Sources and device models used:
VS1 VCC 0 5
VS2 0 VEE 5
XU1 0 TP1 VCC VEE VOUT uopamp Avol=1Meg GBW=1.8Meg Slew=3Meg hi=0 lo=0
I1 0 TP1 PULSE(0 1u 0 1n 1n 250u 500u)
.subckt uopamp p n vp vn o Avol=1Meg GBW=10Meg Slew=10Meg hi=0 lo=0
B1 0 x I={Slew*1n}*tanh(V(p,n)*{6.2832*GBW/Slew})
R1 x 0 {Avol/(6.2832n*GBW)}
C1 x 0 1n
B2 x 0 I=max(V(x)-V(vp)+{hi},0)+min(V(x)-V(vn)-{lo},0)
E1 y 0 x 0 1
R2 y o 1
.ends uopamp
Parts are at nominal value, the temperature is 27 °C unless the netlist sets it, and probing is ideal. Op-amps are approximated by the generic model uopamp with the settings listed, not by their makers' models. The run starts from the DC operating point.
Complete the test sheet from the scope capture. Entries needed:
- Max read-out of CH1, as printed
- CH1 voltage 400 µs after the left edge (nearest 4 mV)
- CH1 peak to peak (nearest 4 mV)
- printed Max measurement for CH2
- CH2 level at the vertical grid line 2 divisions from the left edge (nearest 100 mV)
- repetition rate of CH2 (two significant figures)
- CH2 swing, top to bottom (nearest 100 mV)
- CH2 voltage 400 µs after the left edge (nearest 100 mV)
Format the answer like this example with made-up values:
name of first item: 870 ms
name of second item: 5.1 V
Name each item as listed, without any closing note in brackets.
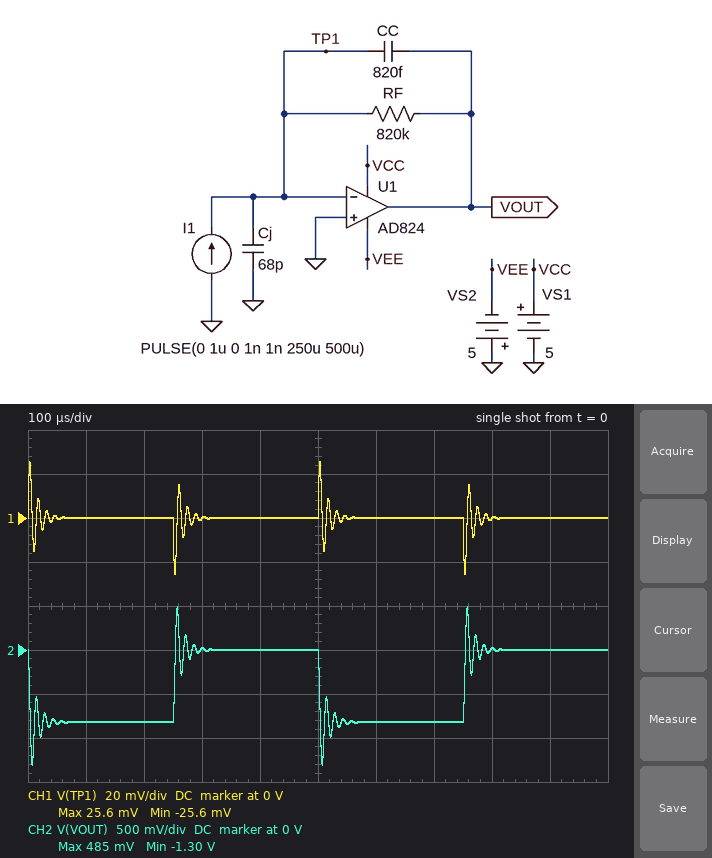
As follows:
Max read-out of CH1, as printed: 25.6 mV
CH1 voltage 400 µs after the left edge: 0 V
CH1 peak to peak: 52 mV
printed Max measurement for CH2: 485 mV
CH2 level at the vertical grid line 2 divisions from the left edge: -800 mV
repetition rate of CH2: 2.0 kHz
CH2 swing, top to bottom: 1.8 V
CH2 voltage 400 µs after the left edge: 0 V
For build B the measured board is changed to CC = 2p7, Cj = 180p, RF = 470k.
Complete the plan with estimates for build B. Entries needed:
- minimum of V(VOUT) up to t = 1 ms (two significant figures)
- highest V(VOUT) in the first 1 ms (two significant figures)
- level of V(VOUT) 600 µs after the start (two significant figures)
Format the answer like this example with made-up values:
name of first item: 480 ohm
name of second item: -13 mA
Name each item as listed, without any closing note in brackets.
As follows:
minimum of V(VOUT) up to t = 1 ms: -680 mV
highest V(VOUT) in the first 1 ms: 210 mV
level of V(VOUT) 600 µs after the start: -470 mV
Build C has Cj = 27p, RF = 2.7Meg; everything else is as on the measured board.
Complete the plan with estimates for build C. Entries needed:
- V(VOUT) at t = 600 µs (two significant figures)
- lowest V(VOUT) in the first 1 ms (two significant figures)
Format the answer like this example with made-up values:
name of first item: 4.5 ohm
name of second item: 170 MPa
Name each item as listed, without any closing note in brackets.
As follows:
V(VOUT) at t = 600 µs: -2.7 V
lowest V(VOUT) in the first 1 ms: -3.3 V
